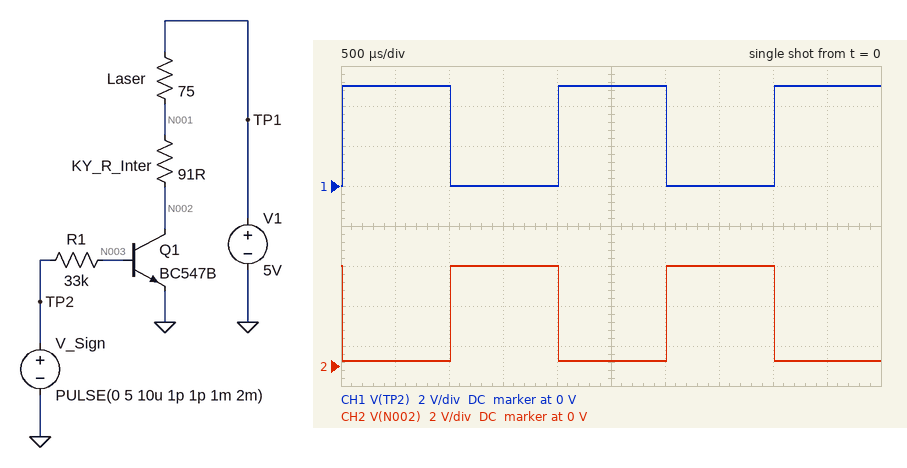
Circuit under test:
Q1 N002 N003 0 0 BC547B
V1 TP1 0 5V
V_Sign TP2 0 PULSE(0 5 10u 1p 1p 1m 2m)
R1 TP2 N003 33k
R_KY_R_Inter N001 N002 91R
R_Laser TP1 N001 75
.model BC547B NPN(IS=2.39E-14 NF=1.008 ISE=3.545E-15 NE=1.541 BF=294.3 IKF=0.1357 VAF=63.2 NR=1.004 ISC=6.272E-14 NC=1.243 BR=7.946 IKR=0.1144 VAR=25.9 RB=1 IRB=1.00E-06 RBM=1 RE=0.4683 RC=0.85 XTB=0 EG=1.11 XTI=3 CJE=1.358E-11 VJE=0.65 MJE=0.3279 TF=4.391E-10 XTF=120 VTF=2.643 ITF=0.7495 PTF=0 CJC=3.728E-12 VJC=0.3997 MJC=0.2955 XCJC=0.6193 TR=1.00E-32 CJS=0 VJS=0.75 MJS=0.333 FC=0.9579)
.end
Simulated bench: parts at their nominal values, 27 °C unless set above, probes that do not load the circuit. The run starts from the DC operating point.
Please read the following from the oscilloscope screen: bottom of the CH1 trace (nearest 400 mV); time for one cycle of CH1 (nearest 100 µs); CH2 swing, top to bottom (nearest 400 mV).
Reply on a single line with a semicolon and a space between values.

0 V; 2.0 ms; 4.8 V
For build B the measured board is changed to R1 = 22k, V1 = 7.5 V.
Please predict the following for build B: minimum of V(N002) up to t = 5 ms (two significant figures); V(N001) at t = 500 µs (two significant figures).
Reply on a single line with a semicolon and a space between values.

600 mV; 4.4 V
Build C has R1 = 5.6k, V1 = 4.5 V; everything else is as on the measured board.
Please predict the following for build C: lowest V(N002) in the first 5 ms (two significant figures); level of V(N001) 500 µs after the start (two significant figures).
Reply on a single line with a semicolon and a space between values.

95 mV; 2.5 V
